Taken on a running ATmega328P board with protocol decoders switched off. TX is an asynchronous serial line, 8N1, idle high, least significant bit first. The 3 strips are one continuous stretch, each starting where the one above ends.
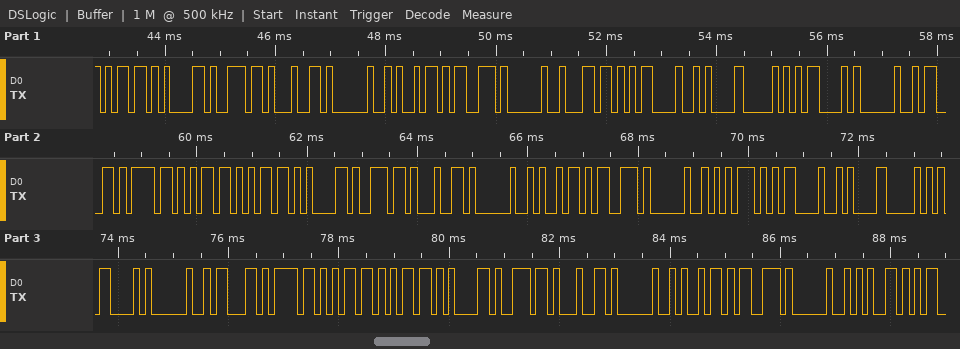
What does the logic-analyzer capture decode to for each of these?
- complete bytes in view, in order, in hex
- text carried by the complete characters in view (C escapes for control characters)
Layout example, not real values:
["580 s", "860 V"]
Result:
["6D 61 6E 64 20 69 73 20 6C 0D 0A 50 43 20 63 6F 6D 6D 61 6E 64 20 69 73 20 75 0D 0A 50 43 20 63 6F 6D 6D 61 6E 64 20 69 73 20 65", "\"mand is l\\r\\nPC command is u\\r\\nPC command is e\""]
